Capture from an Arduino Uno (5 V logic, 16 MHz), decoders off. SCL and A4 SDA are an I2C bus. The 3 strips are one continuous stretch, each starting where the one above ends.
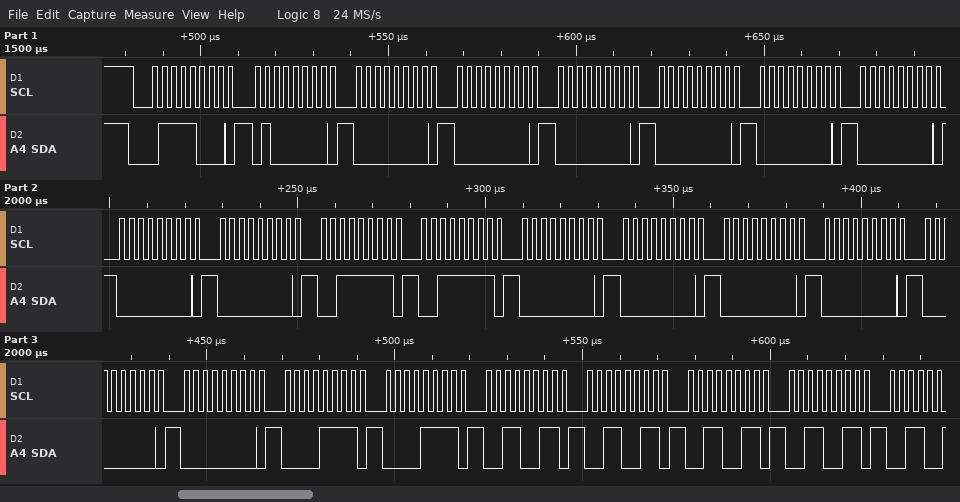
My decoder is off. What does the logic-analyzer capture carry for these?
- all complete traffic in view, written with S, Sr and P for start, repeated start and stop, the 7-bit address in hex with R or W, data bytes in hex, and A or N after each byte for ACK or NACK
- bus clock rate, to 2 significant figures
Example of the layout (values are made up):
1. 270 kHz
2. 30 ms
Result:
1. S 3CW A 40 A 00 A 00 A 00 A 00 A 00 A 00 A 00 A 00 A 3F A 3F A 00 A 00 A 00 A 00 A 00 A 00 A 0F A 0F A 33 A 33 A 33 A 33 A
2. 400 kHz
